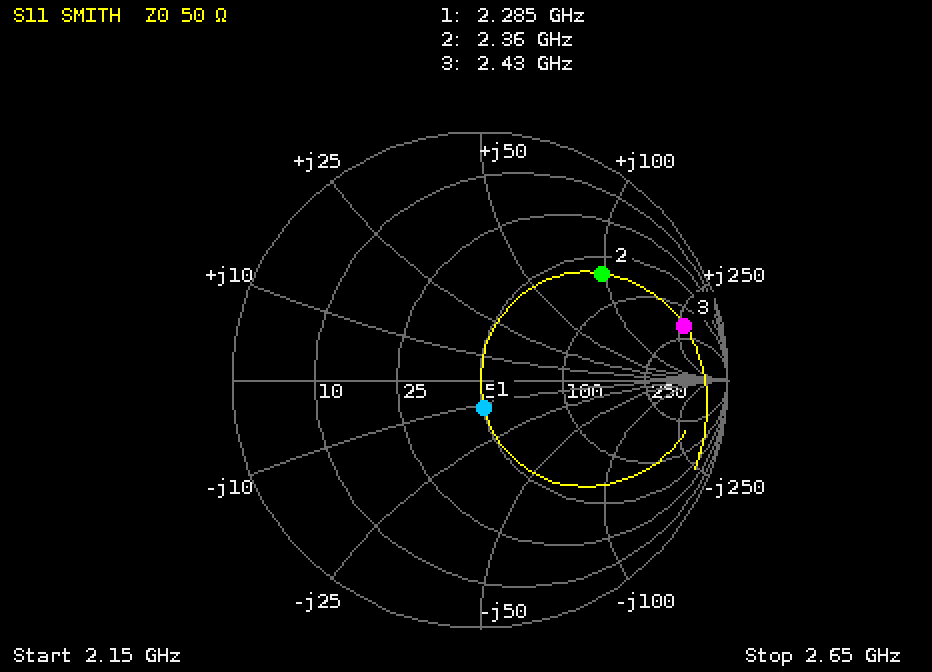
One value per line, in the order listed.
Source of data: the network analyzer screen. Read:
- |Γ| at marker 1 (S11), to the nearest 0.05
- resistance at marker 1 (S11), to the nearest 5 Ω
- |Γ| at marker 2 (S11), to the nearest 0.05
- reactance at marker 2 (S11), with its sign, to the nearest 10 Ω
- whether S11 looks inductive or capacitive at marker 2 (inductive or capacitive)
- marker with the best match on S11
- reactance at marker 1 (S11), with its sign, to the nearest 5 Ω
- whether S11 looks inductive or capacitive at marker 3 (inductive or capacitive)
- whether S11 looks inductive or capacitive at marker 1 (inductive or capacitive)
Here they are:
0.10
50 Ω
0.65
+100 Ω
inductive
marker 1
-10 Ω
inductive
capacitive
